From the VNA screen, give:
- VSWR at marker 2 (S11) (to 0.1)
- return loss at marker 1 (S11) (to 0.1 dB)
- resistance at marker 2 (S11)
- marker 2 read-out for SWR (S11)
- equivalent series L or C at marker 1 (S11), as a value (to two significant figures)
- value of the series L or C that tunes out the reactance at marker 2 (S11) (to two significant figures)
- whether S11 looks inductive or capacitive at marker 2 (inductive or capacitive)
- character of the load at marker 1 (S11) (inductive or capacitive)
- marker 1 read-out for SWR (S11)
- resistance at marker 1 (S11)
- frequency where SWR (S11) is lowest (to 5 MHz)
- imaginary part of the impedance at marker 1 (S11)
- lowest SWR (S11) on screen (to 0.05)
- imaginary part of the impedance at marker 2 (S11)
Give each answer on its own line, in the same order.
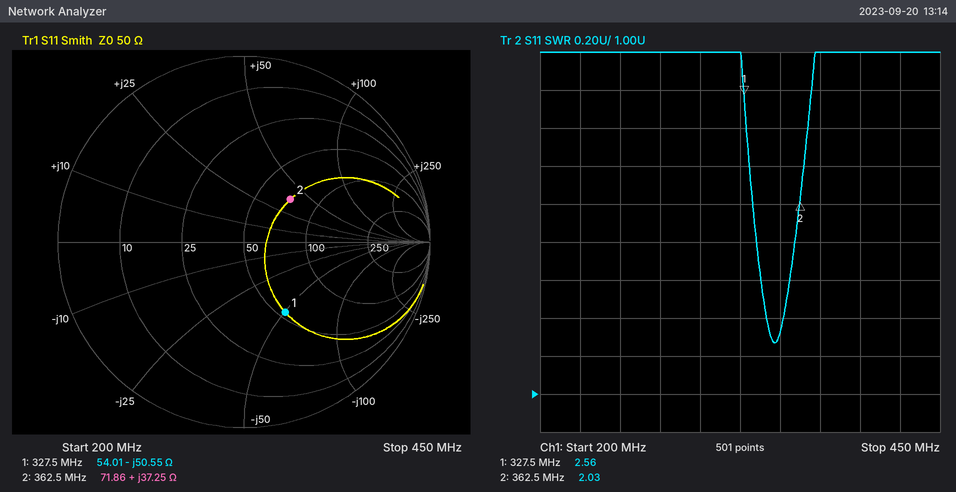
2.0
7.2 dB
71.86 Ω
2.03
9.6 pF
12 pF
inductive
capacitive
2.56
54.01 Ω
345 MHz
-50.55 Ω
1.25
+37.25 Ω
